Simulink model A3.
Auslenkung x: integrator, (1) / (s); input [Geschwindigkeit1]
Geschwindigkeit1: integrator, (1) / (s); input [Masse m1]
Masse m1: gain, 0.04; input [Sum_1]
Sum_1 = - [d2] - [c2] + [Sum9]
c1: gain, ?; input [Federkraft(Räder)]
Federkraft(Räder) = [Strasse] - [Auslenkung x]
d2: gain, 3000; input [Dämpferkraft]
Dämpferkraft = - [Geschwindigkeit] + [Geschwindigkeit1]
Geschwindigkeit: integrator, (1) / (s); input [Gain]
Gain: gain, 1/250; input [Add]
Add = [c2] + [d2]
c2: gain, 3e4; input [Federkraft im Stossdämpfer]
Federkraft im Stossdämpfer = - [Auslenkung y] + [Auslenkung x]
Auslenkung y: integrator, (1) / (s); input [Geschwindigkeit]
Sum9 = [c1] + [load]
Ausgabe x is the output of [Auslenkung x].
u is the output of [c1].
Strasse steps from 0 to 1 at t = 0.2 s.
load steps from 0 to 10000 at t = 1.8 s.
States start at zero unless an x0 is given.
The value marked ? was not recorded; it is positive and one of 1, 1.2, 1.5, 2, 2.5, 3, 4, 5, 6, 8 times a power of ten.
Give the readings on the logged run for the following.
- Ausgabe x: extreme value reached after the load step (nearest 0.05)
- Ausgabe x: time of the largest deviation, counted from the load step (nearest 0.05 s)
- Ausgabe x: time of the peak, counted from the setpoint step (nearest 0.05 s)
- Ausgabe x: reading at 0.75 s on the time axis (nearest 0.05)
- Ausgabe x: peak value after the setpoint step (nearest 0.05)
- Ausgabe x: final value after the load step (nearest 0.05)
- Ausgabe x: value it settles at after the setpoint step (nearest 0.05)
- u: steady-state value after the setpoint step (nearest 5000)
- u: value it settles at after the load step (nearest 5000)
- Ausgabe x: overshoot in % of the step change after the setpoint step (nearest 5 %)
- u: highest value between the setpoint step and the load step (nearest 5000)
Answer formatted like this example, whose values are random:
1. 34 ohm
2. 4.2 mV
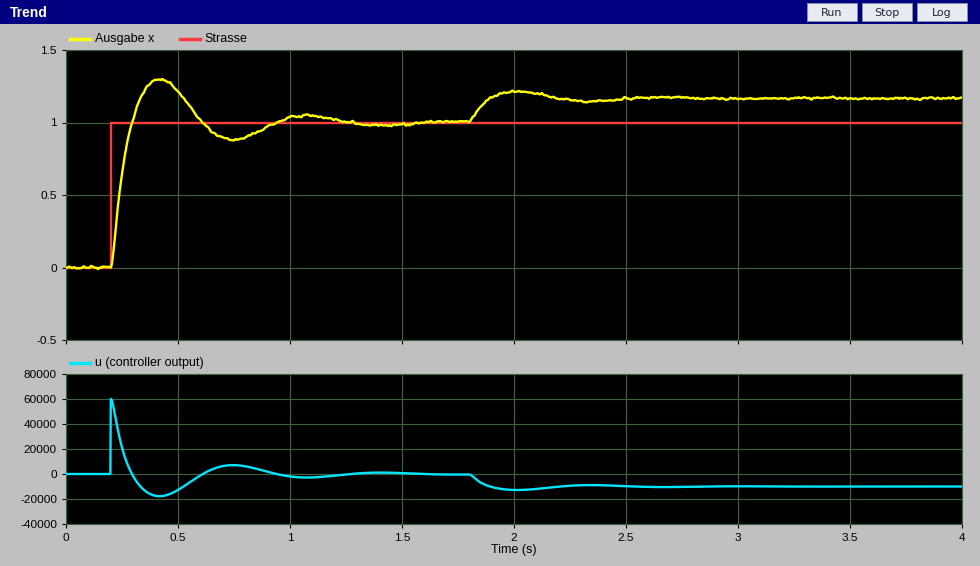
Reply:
1. 1.20
2. 0.20 s
3. 0.20 s
4. 0.90
5. 1.30
6. 1.15
7. 1.00
8. 0
9. -10000
10. 30 %
11. 60000
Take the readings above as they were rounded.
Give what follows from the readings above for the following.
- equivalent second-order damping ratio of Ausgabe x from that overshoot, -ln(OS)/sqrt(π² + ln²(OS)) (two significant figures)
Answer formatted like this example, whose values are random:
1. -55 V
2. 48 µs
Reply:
1. 0.36
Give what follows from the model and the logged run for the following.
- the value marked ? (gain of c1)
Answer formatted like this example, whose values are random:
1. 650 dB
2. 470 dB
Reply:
1. 60000
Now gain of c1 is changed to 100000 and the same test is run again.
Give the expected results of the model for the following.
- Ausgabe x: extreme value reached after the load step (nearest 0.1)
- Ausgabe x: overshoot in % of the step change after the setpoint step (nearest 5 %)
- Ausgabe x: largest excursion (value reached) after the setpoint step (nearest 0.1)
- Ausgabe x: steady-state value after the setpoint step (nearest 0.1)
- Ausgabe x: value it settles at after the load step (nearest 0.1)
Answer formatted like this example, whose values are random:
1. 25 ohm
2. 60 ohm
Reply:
1. 1.1
2. 20 %
3. 1.2
4. 1.0
5. 1.1
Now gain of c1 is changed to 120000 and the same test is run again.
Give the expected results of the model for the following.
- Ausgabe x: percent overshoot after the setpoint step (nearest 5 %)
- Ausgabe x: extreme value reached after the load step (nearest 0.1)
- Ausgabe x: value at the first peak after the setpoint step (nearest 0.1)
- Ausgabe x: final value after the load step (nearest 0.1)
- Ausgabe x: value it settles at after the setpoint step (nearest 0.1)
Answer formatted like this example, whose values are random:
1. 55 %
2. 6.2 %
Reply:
1. 15 %
2. 1.1
3. 1.2
4. 1.1
5. 1.0
